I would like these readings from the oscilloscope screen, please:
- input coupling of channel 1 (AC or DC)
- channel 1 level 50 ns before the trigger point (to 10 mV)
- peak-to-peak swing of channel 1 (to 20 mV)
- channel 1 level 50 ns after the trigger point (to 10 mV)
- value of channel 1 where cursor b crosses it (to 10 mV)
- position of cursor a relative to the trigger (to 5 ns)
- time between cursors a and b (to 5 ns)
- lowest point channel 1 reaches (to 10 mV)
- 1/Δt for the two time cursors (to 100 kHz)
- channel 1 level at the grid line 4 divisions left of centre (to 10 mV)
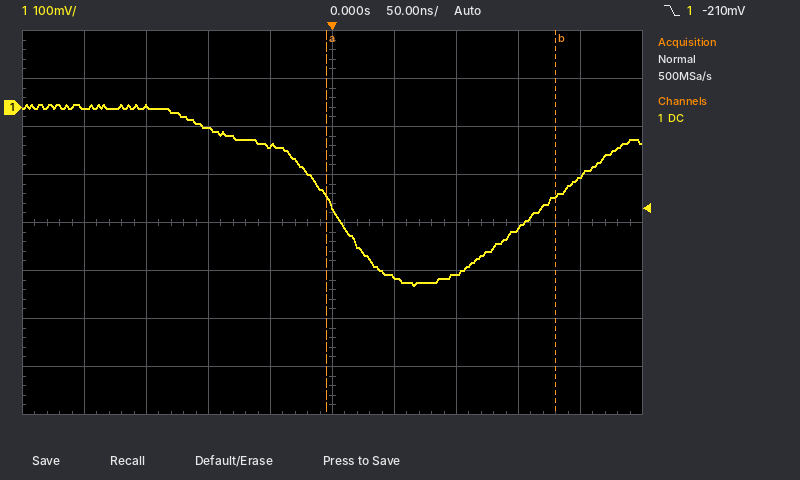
DC
-80 mV
380 mV
-350 mV
-180 mV
-5 ns
185 ns
-370 mV
5.4 MHz
0 mV
